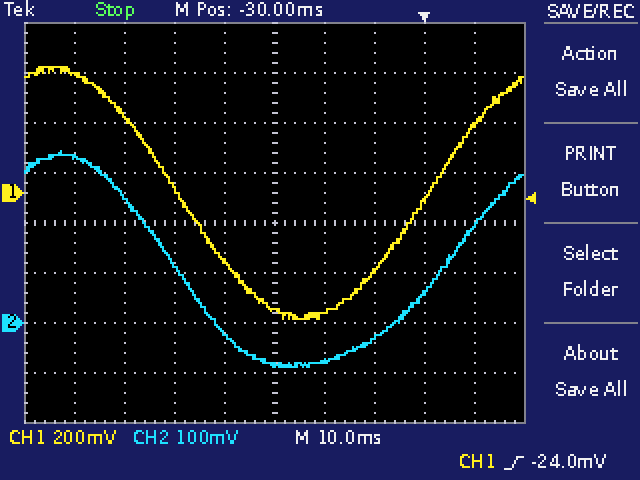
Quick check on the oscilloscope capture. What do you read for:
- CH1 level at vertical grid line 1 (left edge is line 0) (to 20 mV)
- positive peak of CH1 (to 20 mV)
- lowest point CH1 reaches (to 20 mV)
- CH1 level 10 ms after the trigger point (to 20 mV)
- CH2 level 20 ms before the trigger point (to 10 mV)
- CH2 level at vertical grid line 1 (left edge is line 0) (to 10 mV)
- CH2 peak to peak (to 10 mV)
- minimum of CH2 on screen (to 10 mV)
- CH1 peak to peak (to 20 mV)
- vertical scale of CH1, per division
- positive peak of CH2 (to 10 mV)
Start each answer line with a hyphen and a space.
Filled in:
- 480 mV
- 500 mV
- -500 mV
- 280 mV
- -80 mV
- 330 mV
- 430 mV
- -90 mV
- 1.00 V
- 200 mV
- 340 mV
